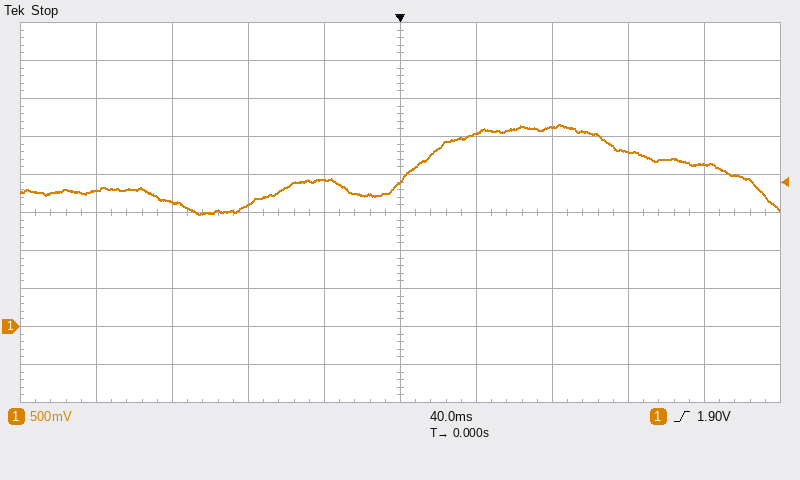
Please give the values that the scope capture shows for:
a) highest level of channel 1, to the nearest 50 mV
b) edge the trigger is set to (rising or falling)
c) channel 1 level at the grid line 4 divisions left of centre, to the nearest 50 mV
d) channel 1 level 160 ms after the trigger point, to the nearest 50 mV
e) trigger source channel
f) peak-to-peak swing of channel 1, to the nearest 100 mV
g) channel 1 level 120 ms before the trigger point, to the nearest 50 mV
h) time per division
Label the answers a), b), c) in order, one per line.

a) 2.65 V
b) rising
c) 1.80 V
d) 2.15 V
e) channel 1
f) 1.20 V
g) 1.65 V
h) 40 ms
